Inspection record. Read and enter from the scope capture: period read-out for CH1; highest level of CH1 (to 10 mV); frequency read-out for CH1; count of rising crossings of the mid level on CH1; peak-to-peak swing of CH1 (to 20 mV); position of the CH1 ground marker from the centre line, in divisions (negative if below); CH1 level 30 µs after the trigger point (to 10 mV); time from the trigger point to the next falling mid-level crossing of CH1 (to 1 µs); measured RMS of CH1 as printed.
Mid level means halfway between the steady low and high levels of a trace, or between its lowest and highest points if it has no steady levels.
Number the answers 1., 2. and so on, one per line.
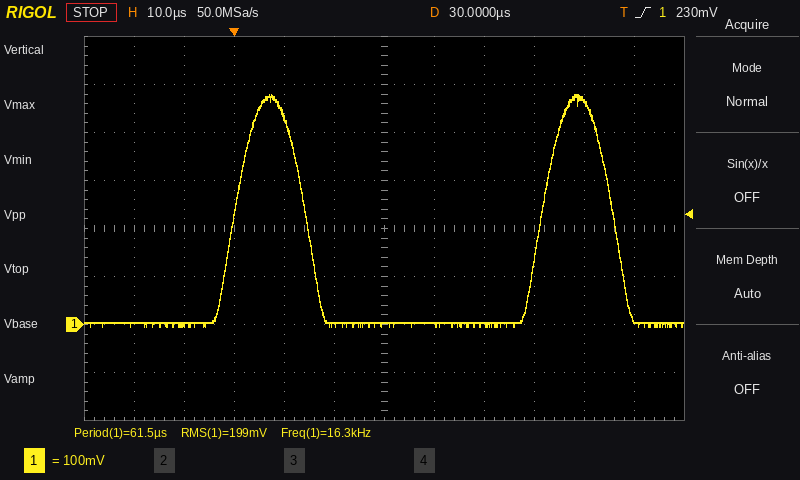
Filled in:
1. 61.5 µs
2. 480 mV
3. 16.3 kHz
4. 2
5. 480 mV
6. -2.0 div
7. 0 mV
8. 14 µs
9. 199 mV
